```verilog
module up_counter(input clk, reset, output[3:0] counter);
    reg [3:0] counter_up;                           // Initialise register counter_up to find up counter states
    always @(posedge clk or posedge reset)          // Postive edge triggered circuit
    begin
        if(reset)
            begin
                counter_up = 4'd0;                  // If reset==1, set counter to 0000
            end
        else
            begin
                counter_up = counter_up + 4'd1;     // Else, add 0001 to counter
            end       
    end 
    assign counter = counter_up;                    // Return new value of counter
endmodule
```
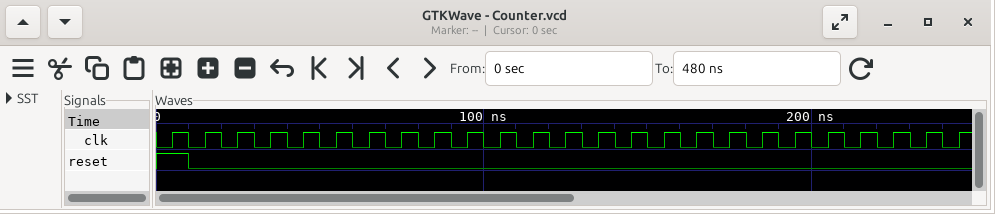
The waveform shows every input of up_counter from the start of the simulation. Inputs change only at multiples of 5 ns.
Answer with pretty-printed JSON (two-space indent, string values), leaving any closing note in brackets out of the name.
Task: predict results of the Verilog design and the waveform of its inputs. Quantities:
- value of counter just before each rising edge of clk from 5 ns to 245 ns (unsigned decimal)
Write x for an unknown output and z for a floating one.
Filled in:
{
  "value of counter just before each rising edge of clk from 5 ns to 245 ns": "0, 0, 1, 2, 3, 4, 5, 6, 7, 8, 9, 10, 11, 12, 13, 14, 15, 0, 1, 2, 3, 4, 5, 6, 7"
}
